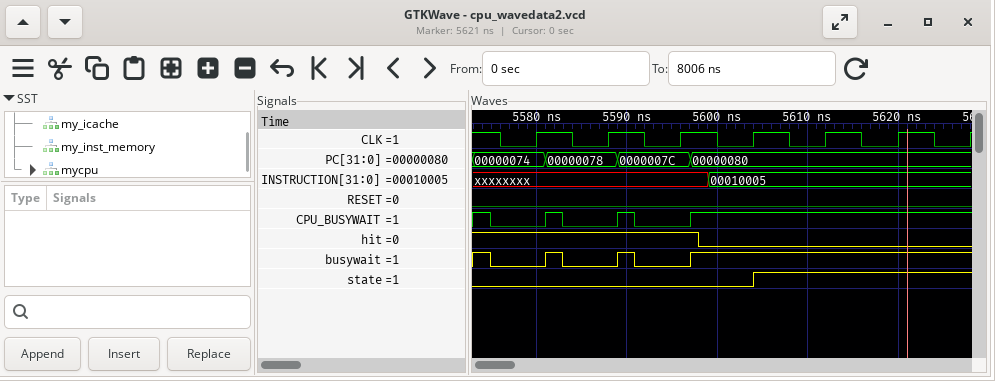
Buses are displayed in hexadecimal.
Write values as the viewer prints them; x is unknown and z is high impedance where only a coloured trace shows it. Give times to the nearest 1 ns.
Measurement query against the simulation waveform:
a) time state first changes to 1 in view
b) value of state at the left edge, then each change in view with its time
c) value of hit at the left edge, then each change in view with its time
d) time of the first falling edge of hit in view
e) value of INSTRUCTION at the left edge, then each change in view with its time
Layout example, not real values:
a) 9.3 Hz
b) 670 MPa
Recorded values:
a) 5604 ns
b) 0, 1 at 5604 ns
c) 1, 0 at 5598 ns
d) 5598 ns
e) xxxxxxxx, 00010005 at 5599 ns
